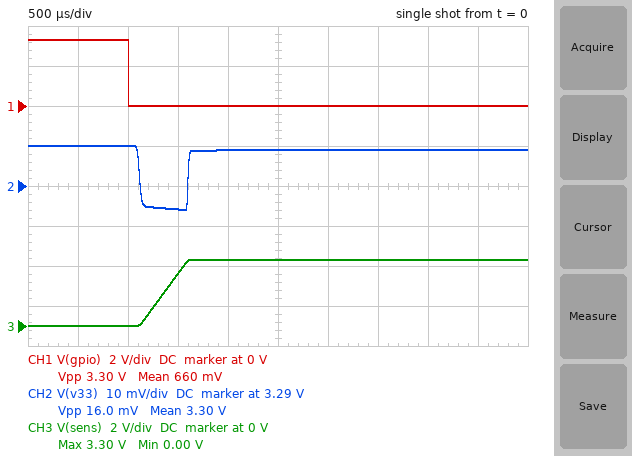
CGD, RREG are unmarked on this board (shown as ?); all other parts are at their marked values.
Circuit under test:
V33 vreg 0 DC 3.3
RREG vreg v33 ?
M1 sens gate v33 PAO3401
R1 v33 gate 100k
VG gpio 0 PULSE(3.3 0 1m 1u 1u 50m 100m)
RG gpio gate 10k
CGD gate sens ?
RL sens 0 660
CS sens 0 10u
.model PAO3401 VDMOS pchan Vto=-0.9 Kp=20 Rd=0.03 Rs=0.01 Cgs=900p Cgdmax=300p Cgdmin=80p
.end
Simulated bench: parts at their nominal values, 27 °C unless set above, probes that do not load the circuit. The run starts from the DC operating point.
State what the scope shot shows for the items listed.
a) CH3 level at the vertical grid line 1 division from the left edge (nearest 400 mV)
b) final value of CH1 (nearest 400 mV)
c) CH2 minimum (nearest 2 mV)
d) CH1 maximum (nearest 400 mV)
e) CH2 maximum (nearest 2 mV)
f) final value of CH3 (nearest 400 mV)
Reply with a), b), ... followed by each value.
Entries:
a) 0 V
b) 0 V
c) 3.284 V
d) 3.2 V
e) 3.300 V
f) 3.2 V
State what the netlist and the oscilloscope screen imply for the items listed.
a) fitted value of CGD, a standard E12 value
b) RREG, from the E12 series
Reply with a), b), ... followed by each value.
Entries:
a) 33 nF
b) 0.22 Ω
